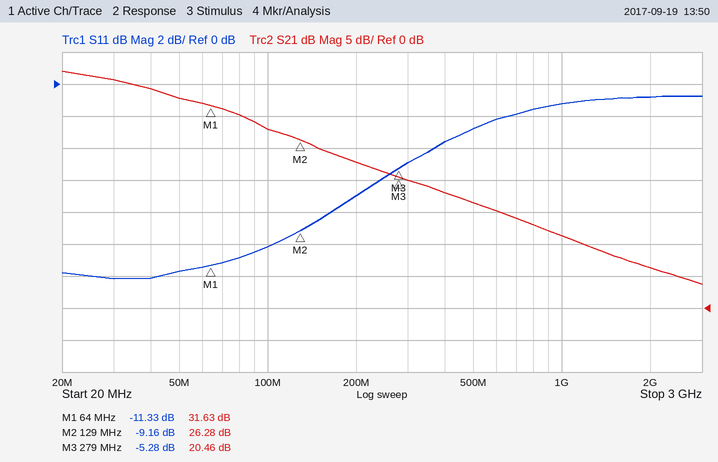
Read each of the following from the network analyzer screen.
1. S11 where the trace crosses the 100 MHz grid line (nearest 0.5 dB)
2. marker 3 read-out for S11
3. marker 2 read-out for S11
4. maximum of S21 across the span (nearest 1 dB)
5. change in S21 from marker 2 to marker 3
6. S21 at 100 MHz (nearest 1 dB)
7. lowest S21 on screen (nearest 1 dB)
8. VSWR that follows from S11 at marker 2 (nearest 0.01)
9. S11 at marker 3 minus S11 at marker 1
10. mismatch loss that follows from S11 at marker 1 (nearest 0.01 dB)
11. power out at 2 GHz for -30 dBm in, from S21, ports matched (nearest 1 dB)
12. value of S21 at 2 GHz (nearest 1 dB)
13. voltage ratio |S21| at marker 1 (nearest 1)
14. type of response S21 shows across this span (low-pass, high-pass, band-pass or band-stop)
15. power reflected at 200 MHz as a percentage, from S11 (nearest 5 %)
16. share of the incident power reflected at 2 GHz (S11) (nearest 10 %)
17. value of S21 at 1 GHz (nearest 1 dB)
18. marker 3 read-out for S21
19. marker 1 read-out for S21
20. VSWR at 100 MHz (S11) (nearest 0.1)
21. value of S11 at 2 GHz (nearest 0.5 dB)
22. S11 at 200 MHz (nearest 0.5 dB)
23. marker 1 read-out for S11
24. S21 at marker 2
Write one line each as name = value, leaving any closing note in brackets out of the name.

S11 where the trace crosses the 100 MHz grid line = -10.0 dB
marker 3 read-out for S11 = -5.28 dB
marker 2 read-out for S11 = -9.16 dB
maximum of S21 across the span = 37 dB
change in S21 from marker 2 to marker 3 = -5.82 dB
S21 at 100 MHz = 28 dB
lowest S21 on screen = 4 dB
VSWR that follows from S11 at marker 2 = 2.07
S11 at marker 3 minus S11 at marker 1 = 6.05 dB
mismatch loss that follows from S11 at marker 1 = 0.33 dB
power out at 2 GHz for -30 dBm in, from S21, ports matched = -24 dBm
value of S21 at 2 GHz = 6 dB
voltage ratio |S21| at marker 1 = 38
type of response S21 shows across this span = low-pass
power reflected at 200 MHz as a percentage, from S11 = 20 %
share of the incident power reflected at 2 GHz (S11) = 80 %
value of S21 at 1 GHz = 11 dB
marker 3 read-out for S21 = 20.46 dB
marker 1 read-out for S21 = 31.63 dB
VSWR at 100 MHz (S11) = 1.9
value of S11 at 2 GHz = -1.0 dB
S11 at 200 MHz = -7.0 dB
marker 1 read-out for S11 = -11.33 dB
S21 at marker 2 = 26.28 dB
